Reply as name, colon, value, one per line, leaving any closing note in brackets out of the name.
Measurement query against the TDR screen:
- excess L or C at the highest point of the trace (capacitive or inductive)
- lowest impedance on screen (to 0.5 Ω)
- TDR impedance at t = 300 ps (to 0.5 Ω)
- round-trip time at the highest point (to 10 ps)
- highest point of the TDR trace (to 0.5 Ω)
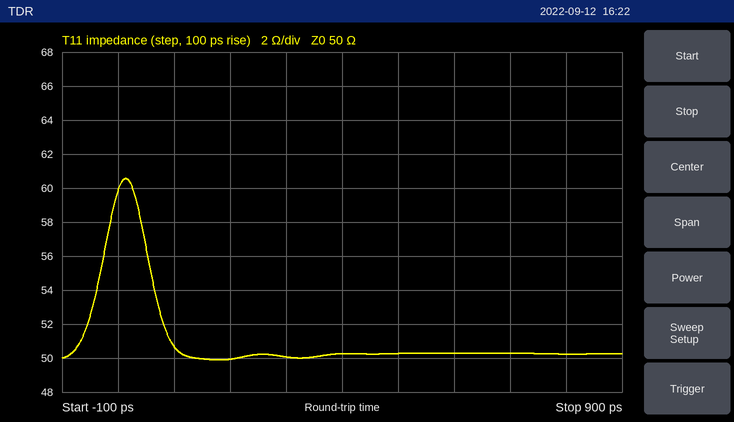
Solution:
excess L or C at the highest point of the trace: inductive
lowest impedance on screen: 50.0 Ω
TDR impedance at t = 300 ps: 50.0 Ω
round-trip time at the highest point: 10 ps
highest point of the TDR trace: 60.5 Ω
